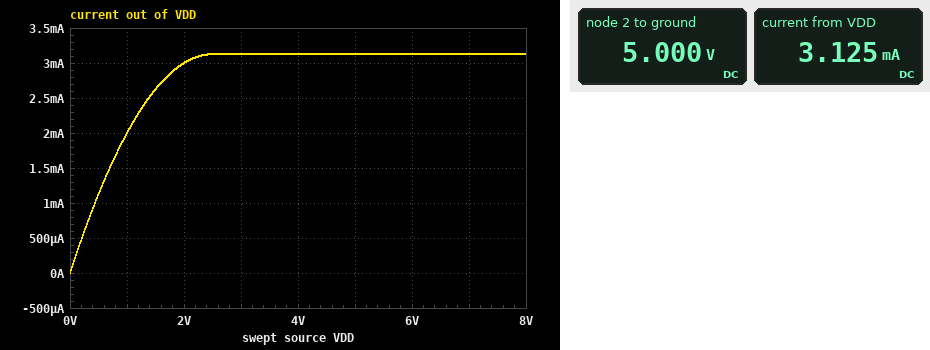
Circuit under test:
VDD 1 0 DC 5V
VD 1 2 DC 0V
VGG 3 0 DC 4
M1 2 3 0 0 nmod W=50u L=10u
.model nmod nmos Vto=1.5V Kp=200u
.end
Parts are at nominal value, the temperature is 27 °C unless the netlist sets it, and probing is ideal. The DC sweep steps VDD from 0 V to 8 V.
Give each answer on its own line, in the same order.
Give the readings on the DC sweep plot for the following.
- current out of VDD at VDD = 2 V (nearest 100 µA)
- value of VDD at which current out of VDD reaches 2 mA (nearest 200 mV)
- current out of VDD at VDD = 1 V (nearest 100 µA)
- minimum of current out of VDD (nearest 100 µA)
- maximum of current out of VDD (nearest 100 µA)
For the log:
3.0 mA
1.0 V
2.0 mA
0 A
3.1 mA
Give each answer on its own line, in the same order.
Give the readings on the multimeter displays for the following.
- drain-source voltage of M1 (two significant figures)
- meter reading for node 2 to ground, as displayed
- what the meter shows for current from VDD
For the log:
5.0 V
5.000 V
3.125 mA
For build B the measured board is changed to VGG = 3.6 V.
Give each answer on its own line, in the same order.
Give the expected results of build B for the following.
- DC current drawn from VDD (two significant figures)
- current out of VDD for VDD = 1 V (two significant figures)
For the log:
2.2 mA
1.6 mA
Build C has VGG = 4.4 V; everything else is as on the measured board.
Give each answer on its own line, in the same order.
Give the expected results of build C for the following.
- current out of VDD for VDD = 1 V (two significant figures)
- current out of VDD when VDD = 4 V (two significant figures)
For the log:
2.4 mA
4.2 mA
